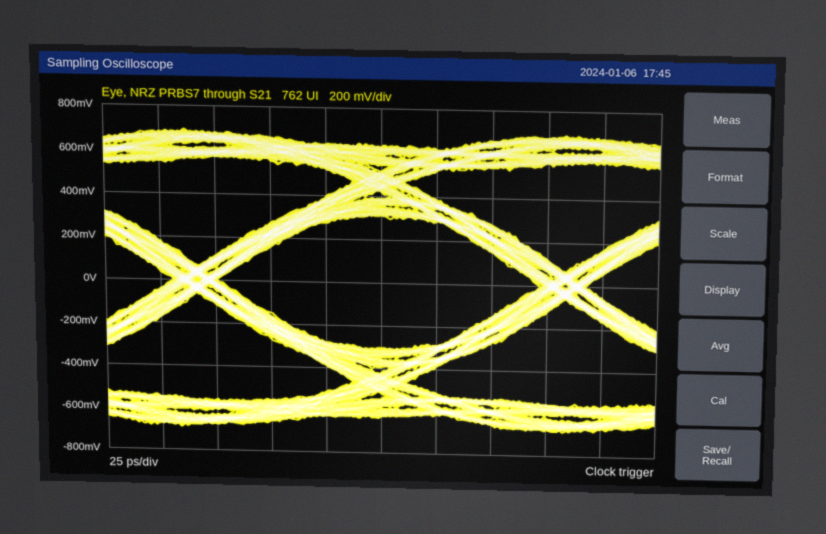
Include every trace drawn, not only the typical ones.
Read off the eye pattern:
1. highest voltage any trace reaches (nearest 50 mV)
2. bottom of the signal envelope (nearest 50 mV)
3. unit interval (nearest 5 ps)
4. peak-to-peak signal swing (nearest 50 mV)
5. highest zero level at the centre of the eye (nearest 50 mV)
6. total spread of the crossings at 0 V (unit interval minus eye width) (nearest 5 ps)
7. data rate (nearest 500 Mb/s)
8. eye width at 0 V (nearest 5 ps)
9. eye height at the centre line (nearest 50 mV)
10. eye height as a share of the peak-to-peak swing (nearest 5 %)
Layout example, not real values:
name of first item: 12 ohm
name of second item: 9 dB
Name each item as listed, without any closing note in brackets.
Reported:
highest voltage any trace reaches: 700 mV
bottom of the signal envelope: -700 mV
unit interval: 165 ps
peak-to-peak signal swing: 1.40 V
highest zero level at the centre of the eye: -300 mV
total spread of the crossings at 0 V (unit interval minus eye width): 20 ps
data rate: 6.0 Gb/s
eye width at 0 V: 145 ps
eye height at the centre line: 600 mV
eye height as a share of the peak-to-peak swing: 45 %
